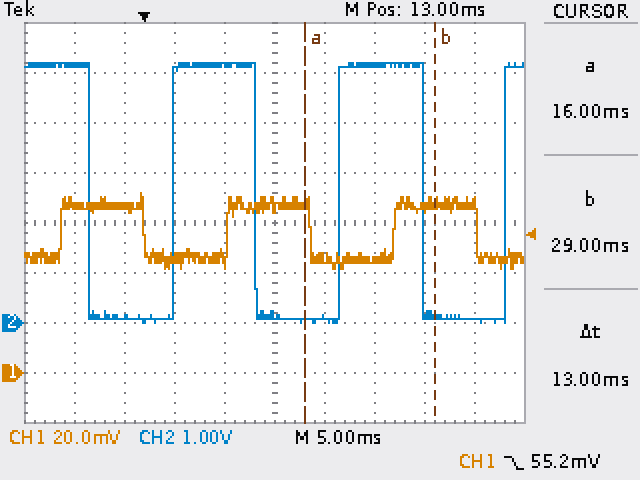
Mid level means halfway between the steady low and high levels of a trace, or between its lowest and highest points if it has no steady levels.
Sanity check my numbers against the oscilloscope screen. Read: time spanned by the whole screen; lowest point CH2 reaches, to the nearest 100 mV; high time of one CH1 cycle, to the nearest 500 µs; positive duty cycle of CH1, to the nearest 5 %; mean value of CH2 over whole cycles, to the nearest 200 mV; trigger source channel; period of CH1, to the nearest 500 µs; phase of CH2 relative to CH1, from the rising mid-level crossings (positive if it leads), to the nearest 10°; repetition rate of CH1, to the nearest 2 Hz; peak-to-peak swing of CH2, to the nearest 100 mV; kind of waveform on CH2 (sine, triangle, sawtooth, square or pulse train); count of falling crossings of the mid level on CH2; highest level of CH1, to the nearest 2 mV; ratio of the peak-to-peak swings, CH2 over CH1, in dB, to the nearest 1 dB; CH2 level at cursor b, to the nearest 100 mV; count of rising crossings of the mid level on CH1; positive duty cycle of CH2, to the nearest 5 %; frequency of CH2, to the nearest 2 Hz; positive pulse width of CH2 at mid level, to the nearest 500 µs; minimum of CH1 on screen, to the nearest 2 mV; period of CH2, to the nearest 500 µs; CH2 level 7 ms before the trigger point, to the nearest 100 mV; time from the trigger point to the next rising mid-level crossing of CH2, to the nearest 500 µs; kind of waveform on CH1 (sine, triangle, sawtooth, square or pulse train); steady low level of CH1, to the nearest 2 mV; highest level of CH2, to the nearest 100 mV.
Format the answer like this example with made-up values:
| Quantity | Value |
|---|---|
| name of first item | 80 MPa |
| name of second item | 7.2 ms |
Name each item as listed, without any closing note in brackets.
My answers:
| Quantity | Value |
|---|---|
| time spanned by the whole screen | 50 ms |
| lowest point CH2 reaches, to the nearest 100 mV | 0.0 V |
| high time of one CH1 cycle, to the nearest 500 µs | 8.5 ms |
| positive duty cycle of CH1, to the nearest 5 % | 50 % |
| mean value of CH2 over whole cycles, to the nearest 200 mV | 2.6 V |
| trigger source channel | CH1 |
| period of CH1, to the nearest 500 µs | 16.5 ms |
| phase of CH2 relative to CH1, from the rising mid-level crossings (positive if it leads), to the nearest 10° | +120° |
| repetition rate of CH1, to the nearest 2 Hz | 60 Hz |
| peak-to-peak swing of CH2, to the nearest 100 mV | 5.2 V |
| kind of waveform on CH2 | square |
| count of falling crossings of the mid level on CH2 | 3 |
| highest level of CH1, to the nearest 2 mV | 72 mV |
| ratio of the peak-to-peak swings, CH2 over CH1, in dB, to the nearest 1 dB | 45 dB |
| CH2 level at cursor b, to the nearest 100 mV | 200 mV |
| count of rising crossings of the mid level on CH1 | 3 |
| positive duty cycle of CH2, to the nearest 5 % | 50 % |
| frequency of CH2, to the nearest 2 Hz | 60 Hz |
| positive pulse width of CH2 at mid level, to the nearest 500 µs | 8.5 ms |
| minimum of CH1 on screen, to the nearest 2 mV | 42 mV |
| period of CH2, to the nearest 500 µs | 16.5 ms |
| CH2 level 7 ms before the trigger point, to the nearest 100 mV | 5.2 V |
| time from the trigger point to the next rising mid-level crossing of CH2, to the nearest 500 µs | 3.0 ms |
| kind of waveform on CH1 | square |
| steady low level of CH1, to the nearest 2 mV | 46 mV |
| highest level of CH2, to the nearest 100 mV | 5.2 V |
